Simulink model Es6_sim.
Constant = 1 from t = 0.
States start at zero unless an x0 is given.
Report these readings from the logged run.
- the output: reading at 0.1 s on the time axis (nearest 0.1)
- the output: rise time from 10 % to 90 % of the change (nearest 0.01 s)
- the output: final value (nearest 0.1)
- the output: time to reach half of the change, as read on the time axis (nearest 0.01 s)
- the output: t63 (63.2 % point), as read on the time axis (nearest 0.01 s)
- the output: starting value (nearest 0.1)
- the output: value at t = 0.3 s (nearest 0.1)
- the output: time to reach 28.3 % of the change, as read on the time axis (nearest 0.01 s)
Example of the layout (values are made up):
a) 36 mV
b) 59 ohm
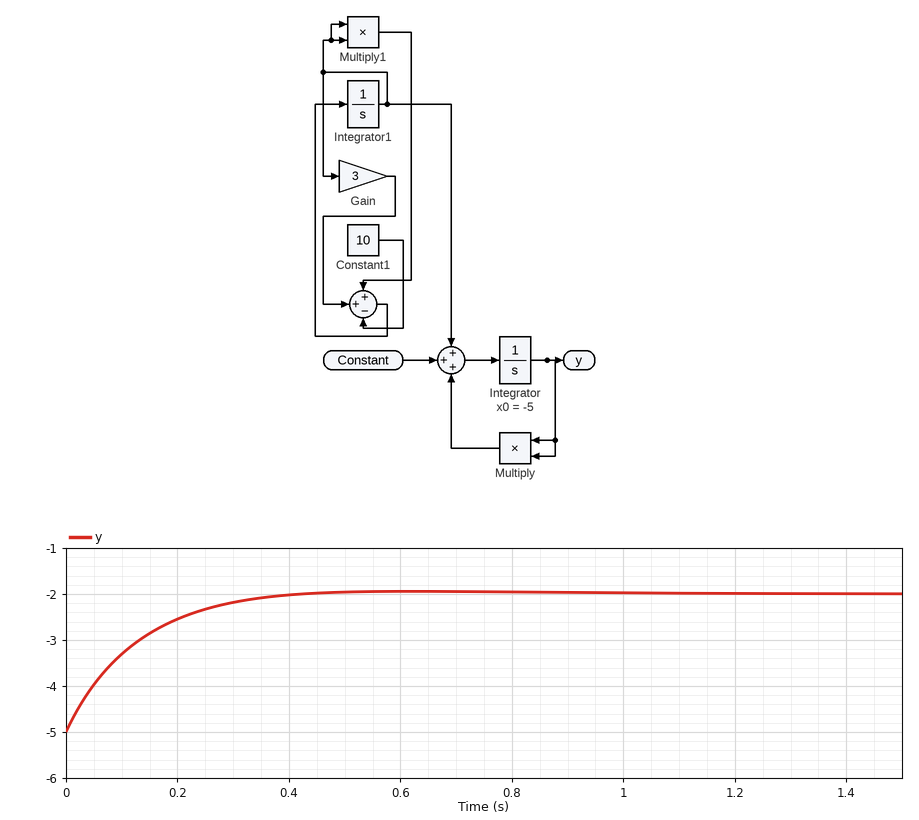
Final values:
a) -3.3
b) 0.25 s
c) -2.0
d) 0.08 s
e) 0.12 s
f) -5.0
g) -2.2
h) 0.04 s
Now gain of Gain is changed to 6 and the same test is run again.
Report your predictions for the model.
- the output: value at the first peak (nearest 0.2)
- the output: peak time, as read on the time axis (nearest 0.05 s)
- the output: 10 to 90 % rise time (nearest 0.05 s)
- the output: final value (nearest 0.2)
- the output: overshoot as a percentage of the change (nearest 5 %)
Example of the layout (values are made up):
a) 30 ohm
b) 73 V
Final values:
a) -2.2
b) 0.40 s
c) 0.15 s
d) -2.6
e) 10 %
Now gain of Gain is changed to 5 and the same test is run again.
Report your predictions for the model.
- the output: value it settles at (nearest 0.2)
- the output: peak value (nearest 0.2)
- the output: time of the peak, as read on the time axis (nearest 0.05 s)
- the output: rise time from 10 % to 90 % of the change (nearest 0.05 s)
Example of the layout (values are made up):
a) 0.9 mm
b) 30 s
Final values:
a) -2.4
b) -2.2
c) 0.45 s
d) 0.20 s
